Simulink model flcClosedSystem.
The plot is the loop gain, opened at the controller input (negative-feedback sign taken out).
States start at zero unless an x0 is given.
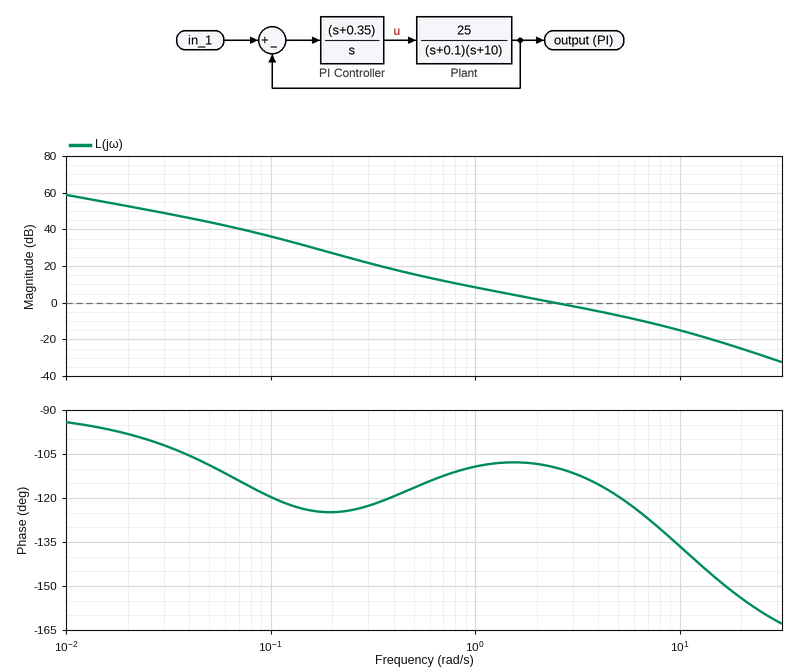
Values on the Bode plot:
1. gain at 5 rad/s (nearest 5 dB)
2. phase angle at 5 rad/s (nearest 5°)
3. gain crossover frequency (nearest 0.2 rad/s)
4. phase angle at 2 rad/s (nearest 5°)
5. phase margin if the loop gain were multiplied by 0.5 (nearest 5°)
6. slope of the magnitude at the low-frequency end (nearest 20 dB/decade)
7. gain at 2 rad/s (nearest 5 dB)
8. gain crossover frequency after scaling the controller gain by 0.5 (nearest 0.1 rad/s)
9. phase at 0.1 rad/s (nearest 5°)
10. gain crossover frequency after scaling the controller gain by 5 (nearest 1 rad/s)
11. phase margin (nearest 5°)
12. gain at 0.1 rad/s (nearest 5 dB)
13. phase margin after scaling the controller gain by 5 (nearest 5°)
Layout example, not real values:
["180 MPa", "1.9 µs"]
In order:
["-5 dB", "-120°", "2.4 rad/s", "-110°", "70°", "-20 dB/decade", "0 dB", "1.3 rad/s", "-120°", "9 rad/s", "70°", "35 dB", "45°"]
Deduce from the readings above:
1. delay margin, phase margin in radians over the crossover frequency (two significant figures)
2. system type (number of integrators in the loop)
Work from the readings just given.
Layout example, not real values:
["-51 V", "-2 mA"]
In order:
["0.51 s", "1"]
